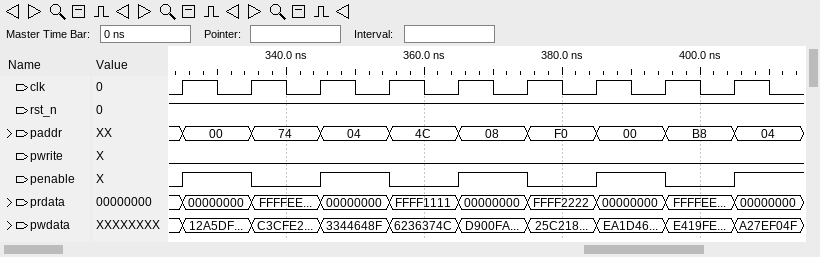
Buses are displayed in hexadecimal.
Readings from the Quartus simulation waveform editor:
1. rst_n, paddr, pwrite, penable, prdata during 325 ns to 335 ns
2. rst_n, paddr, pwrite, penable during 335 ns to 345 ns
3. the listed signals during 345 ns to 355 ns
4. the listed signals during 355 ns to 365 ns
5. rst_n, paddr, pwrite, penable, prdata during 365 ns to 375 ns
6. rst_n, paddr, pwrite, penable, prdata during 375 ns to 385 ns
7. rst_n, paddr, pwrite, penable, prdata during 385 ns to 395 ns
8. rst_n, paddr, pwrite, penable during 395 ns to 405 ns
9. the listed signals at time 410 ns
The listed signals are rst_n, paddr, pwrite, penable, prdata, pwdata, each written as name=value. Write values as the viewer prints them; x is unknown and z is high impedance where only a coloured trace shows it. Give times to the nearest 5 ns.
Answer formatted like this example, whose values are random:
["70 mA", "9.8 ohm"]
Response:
["rst_n=1, paddr=00, pwrite=0, penable=1, prdata=00000000", "rst_n=1, paddr=74, pwrite=0, penable=0", "rst_n=1, paddr=04, pwrite=0, penable=1, prdata=00000000, pwdata=3344648F", "rst_n=1, paddr=4C, pwrite=0, penable=0, prdata=FFFF1111, pwdata=6236374C", "rst_n=1, paddr=08, pwrite=0, penable=1, prdata=00000000", "rst_n=1, paddr=F0, pwrite=0, penable=0, prdata=FFFF2222", "rst_n=1, paddr=00, pwrite=0, penable=1, prdata=00000000", "rst_n=1, paddr=B8, pwrite=0, penable=0", "rst_n=1, paddr=04, pwrite=0, penable=1, prdata=00000000, pwdata=A27EF04F"]
